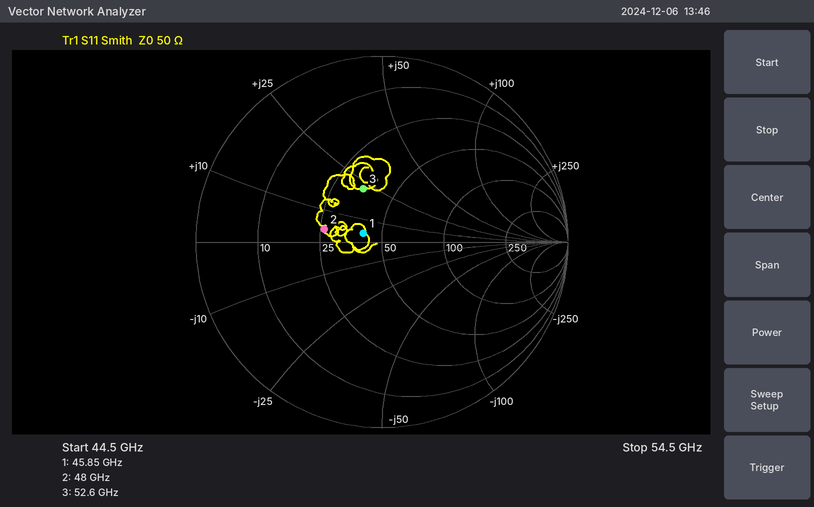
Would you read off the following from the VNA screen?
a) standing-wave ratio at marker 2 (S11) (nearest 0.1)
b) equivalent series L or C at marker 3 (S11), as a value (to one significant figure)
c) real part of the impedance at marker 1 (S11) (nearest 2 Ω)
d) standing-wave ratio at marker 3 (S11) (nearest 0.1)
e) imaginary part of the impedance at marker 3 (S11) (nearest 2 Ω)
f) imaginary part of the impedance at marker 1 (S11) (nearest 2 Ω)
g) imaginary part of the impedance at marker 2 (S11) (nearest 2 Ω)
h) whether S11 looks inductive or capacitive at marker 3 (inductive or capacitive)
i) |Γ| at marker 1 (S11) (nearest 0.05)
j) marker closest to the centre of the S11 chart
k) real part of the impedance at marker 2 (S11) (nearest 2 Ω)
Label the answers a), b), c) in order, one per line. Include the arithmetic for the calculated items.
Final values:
a) 1.9
b) L = 22 Ω/(2π × 52.6 GHz) ≈ 66.6 pH, so 70 pH to one significant figure
c) 40 Ω
d) 1.9
e) +22 Ω
f) +4 Ω
g) +4 Ω
h) inductive
i) 0.10
j) marker 1
k) 26 Ω
